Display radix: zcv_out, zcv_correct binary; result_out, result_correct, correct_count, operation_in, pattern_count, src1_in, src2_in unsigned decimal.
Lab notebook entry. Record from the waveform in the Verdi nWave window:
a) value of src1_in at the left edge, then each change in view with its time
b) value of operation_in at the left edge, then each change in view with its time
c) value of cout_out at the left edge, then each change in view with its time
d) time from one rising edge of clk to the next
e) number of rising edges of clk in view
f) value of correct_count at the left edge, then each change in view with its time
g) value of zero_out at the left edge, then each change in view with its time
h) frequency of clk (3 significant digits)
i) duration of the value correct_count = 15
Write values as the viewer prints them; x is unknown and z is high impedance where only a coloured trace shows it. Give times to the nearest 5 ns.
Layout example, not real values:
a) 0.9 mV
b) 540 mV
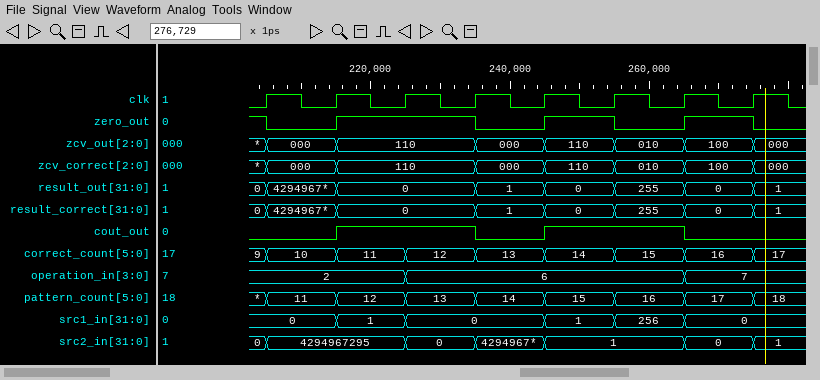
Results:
a) 0, 1 at 215 ns, 0 at 225 ns, 1 at 245 ns, 256 at 255 ns, 0 at 265 ns
b) 2, 6 at 225 ns, 7 at 265 ns
c) 0, 1 at 215 ns, 0 at 235 ns, 1 at 245 ns, 0 at 265 ns
d) 10 ns
e) 8
f) 9, 10 at 205 ns, 11 at 215 ns, 12 at 225 ns, 13 at 235 ns, 14 at 245 ns, 15 at 255 ns, 16 at 265 ns, 17 at 275 ns
g) 1, 0 at 205 ns, 1 at 215 ns, 0 at 235 ns, 1 at 245 ns, 0 at 255 ns, 1 at 265 ns, 0 at 275 ns
h) 100 MHz
i) 10 ns
